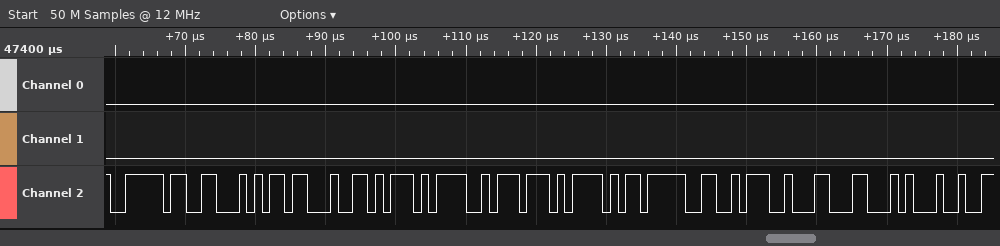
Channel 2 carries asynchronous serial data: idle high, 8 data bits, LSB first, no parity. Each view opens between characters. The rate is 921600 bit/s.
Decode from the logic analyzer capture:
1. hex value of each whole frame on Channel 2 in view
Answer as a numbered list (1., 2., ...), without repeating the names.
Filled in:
1. BE, 46, 1B, D6, 3D, 77, AF, 9F, 3A, 8C, 14
